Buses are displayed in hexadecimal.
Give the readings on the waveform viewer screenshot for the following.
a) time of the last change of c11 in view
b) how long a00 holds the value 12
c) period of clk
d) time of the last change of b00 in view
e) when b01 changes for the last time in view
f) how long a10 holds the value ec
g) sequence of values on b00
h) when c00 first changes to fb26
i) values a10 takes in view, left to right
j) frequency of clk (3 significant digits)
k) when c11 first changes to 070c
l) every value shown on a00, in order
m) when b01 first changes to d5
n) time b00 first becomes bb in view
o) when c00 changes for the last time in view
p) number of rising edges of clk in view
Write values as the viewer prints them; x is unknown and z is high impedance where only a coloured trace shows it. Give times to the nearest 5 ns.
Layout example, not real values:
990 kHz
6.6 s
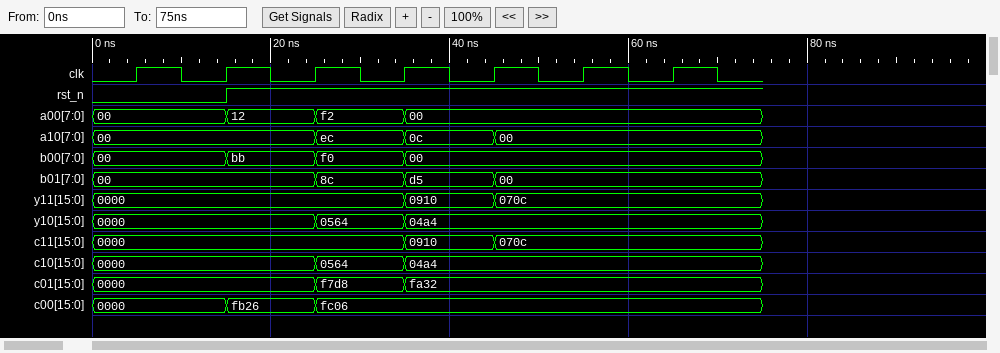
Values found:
45 ns
10 ns
10 ns
35 ns
45 ns
10 ns
00, bb, f0, 00
15 ns
00, ec, 0c, 00
100 MHz
45 ns
00, 12, f2, 00
35 ns
15 ns
25 ns
7
